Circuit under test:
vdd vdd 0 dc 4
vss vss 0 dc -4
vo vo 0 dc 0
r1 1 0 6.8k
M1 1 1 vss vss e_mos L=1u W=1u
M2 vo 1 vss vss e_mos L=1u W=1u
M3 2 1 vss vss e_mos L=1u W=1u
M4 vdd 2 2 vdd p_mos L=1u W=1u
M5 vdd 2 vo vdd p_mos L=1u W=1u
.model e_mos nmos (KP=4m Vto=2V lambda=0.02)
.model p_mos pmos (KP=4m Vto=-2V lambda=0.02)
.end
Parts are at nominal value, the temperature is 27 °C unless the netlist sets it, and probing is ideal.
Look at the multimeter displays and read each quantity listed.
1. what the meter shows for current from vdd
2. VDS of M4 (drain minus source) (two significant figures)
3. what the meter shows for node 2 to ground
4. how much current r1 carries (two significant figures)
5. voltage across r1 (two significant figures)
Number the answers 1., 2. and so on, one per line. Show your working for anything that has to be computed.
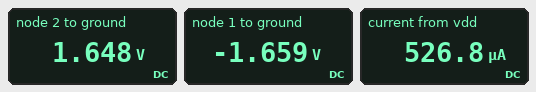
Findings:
1. 526.8 µA
2. 4 V - 1.648 V = 2.4 V
3. 1.648 V
4. (0 V - (-1.659 V)) / 6.8 kΩ = 240 µA
5. 0 V - (-1.659 V) = 1.7 V
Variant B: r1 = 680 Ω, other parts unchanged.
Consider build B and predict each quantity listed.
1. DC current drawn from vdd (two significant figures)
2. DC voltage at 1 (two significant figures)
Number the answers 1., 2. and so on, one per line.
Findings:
1. 3.5 mA
2. -1.1 V
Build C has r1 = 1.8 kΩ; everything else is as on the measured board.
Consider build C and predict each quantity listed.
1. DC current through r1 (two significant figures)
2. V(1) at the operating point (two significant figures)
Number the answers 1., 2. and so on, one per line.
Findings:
1. 770 µA
2. -1.4 V
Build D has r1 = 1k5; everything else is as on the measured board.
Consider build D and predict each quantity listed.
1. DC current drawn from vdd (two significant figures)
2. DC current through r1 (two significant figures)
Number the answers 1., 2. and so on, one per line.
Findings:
1. 1.9 mA
2. 900 µA
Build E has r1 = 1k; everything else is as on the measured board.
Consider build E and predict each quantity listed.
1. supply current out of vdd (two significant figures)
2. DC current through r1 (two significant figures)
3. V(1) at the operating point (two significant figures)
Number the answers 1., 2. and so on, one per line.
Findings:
1. 2.6 mA
2. 1.2 mA
3. -1.2 V
